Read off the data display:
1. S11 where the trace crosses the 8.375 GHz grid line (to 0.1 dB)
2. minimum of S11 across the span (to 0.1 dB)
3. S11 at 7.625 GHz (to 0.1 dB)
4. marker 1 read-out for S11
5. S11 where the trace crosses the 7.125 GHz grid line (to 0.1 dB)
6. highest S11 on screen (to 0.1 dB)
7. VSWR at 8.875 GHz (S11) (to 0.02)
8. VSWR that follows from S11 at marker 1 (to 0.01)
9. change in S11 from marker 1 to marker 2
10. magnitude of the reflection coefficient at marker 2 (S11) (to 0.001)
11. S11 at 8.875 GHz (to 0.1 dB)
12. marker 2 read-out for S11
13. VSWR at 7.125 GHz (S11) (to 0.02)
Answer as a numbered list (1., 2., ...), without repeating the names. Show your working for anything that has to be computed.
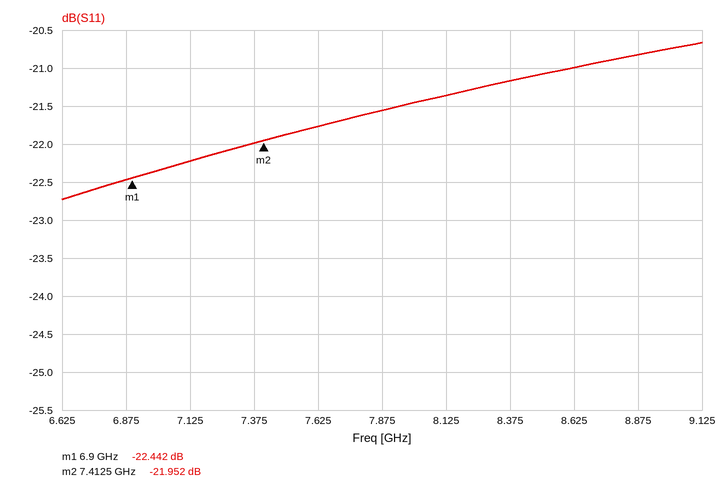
1. -21.2 dB
2. -22.7 dB
3. -21.8 dB
4. -22.442 dB
5. -22.2 dB
6. -20.7 dB
7. |Γ| = 10^(-20.8/20) = 0.0912; VSWR = (1 + 0.0912)/(1 − 0.0912) ≈ 1.20
8. (1 + 0.0755)/(1 − 0.0755) ≈ 1.16
9. -21.952 − (-22.442) = 0.490 dB
10. 10^(-21.952/20) ≈ 0.080
11. -20.8 dB
12. -21.952 dB
13. |Γ| = 10^(-22.2/20) = 0.0776; VSWR = (1 + 0.0776)/(1 − 0.0776) ≈ 1.17, so 1.16 to the nearest 0.02
